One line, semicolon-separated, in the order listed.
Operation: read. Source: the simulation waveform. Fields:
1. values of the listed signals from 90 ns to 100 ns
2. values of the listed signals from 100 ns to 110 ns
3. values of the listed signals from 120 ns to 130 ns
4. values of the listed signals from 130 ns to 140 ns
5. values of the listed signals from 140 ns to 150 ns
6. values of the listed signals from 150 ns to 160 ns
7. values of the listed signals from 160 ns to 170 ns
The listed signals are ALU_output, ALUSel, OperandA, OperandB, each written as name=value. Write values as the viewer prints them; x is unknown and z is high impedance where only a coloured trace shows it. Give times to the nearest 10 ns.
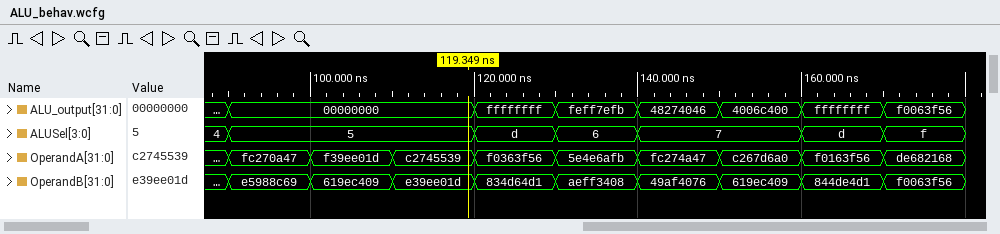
ALU_output=00000000, ALUSel=5, OperandA=fc270a47, OperandB=e5988c69; ALU_output=00000000, ALUSel=5, OperandA=f39ee01d, OperandB=619ec409; ALU_output=ffffffff, ALUSel=d, OperandA=f0363f56, OperandB=834d64d1; ALU_output=feff7efb, ALUSel=6, OperandA=5e4e6afb, OperandB=aeff3408; ALU_output=48274046, ALUSel=7, OperandA=fc274a47, OperandB=49af4076; ALU_output=4006c400, ALUSel=7, OperandA=c267d6a0, OperandB=619ec409; ALU_output=ffffffff, ALUSel=d, OperandA=f0163f56, OperandB=844de4d1
